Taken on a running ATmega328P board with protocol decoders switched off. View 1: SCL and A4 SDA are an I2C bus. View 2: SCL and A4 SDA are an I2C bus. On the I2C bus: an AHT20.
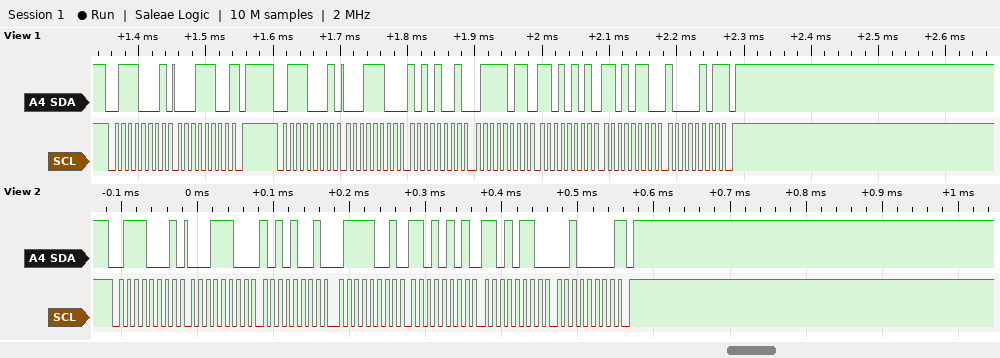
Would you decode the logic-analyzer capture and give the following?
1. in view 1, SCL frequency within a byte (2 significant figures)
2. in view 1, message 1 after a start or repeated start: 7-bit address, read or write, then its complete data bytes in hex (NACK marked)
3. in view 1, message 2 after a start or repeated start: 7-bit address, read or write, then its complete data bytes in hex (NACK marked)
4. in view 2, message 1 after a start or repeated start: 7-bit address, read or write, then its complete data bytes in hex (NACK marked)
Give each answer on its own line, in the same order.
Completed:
100 kHz
0x38 read: 1C NACK
0x38 read: 1C A9 7B D5 D6 85 NACK
0x38 read: 1C A9 79 D5 D6 20 NACK
